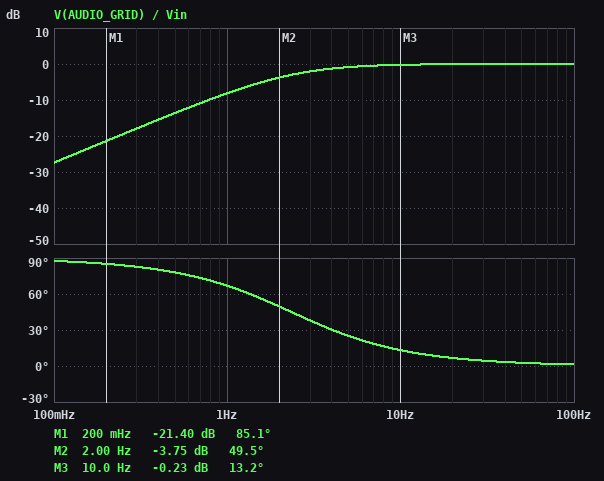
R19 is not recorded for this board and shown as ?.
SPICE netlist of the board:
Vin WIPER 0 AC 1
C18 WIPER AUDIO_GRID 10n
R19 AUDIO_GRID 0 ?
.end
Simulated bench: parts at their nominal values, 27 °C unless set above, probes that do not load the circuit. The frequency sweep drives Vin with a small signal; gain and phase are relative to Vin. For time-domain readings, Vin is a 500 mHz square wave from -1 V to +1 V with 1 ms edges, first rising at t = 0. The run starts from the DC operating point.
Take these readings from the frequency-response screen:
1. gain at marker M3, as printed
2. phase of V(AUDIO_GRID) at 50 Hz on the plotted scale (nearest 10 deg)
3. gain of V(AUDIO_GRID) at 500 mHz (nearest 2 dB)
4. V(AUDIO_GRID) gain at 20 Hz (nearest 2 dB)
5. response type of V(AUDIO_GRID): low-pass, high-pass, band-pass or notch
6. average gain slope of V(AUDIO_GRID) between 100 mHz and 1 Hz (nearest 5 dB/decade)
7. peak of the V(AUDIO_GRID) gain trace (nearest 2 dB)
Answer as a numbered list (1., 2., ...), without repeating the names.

1. -0.23 dB
2. 0 deg
3. -14 dB
4. 0 dB
5. high-pass
6. 20 dB/decade
7. 0 dB
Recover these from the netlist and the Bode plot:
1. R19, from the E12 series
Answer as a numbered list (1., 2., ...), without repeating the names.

1. 6.8 MΩ
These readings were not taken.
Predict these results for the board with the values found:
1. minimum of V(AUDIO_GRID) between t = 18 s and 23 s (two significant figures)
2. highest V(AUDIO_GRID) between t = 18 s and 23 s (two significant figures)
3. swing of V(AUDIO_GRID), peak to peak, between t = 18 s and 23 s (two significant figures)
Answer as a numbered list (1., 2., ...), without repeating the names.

1. -2.0 V
2. 2.0 V
3. 4.0 V
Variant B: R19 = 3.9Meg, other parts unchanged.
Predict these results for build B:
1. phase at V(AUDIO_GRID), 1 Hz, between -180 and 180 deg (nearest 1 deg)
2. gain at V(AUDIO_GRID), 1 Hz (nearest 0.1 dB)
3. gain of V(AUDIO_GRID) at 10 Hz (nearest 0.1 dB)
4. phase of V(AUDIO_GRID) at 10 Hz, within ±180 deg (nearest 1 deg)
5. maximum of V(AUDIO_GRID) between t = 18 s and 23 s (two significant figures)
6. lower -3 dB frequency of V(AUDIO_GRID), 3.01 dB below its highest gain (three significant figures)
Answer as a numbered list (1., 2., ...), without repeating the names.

1. 76 deg
2. -12.5 dB
3. -0.7 dB
4. 22 deg
5. 2.0 V
6. 4.08 Hz
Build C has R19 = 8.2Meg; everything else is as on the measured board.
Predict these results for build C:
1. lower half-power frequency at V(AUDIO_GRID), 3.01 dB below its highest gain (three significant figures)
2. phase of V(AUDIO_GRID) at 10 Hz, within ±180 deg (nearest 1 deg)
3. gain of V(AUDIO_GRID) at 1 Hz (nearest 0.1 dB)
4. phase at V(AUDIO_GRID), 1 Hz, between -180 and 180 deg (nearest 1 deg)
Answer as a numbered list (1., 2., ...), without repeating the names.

1. 1.94 Hz
2. 11 deg
3. -6.8 dB
4. 63 deg
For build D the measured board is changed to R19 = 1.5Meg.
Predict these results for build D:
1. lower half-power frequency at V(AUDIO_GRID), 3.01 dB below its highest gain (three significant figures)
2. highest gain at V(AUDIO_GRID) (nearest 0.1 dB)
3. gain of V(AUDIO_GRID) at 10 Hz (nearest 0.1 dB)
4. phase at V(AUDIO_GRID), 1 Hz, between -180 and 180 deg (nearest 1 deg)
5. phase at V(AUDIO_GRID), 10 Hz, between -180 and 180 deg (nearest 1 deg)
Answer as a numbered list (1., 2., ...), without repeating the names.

1. 10.6 Hz
2. 0 dB
3. -3.3 dB
4. 85 deg
5. 47 deg
